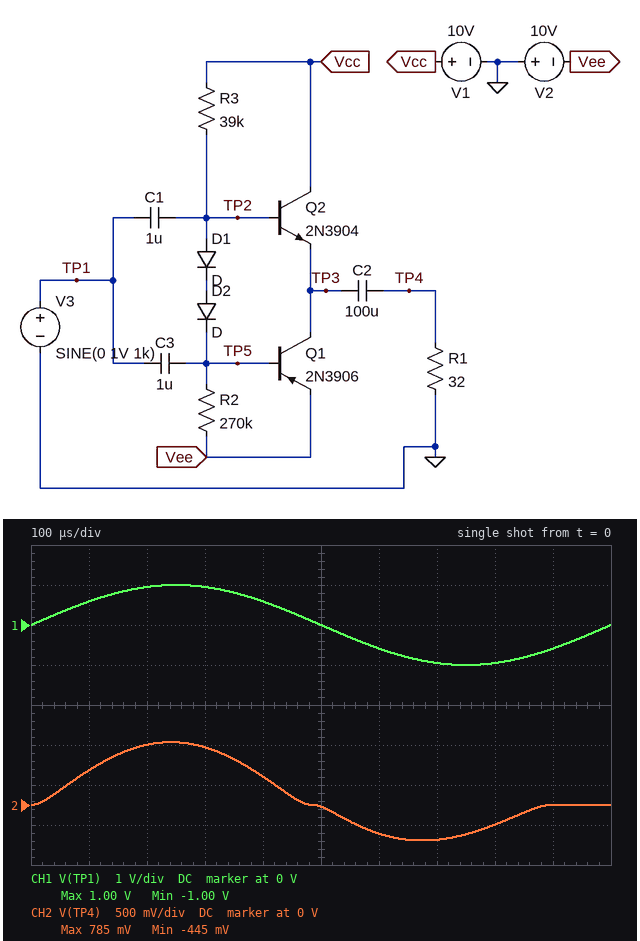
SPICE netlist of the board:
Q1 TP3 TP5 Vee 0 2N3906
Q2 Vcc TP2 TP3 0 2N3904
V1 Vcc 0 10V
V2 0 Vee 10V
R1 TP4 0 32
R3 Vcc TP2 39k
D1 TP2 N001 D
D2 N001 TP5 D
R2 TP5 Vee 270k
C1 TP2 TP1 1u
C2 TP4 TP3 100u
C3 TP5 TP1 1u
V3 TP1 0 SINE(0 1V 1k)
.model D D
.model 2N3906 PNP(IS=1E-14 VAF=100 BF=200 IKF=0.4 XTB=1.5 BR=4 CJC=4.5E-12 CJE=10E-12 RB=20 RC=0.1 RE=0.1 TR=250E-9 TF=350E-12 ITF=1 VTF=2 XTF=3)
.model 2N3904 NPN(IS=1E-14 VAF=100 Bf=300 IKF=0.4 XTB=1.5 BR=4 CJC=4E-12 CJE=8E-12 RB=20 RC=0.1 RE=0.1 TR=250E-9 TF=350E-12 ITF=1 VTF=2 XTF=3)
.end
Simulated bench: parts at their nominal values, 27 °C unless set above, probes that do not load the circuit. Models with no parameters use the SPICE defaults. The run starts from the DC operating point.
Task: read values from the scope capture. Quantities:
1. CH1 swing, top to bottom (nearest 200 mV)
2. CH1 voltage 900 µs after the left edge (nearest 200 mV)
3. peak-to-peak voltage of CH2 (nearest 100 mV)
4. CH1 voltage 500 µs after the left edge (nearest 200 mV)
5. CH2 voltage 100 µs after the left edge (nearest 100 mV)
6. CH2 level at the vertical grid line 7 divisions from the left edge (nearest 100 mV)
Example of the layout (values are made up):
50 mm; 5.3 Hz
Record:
2.0 V; -600 mV; 1.2 V; 0 V; 400 mV; -400 mV
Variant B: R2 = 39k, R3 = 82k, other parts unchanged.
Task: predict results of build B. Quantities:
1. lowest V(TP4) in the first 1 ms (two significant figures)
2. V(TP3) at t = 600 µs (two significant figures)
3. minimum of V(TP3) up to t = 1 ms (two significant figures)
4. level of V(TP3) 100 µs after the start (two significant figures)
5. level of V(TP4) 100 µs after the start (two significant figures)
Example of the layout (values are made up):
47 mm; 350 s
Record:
-470 mV; -2.8 V; -2.9 V; -2.0 V; 460 mV
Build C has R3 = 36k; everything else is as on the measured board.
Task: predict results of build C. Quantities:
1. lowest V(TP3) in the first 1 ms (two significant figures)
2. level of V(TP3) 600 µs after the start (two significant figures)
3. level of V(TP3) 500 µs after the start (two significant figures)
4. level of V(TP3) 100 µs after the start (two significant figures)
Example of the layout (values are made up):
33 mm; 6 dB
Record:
7.2 V; 7.3 V; 7.6 V; 8.0 V
